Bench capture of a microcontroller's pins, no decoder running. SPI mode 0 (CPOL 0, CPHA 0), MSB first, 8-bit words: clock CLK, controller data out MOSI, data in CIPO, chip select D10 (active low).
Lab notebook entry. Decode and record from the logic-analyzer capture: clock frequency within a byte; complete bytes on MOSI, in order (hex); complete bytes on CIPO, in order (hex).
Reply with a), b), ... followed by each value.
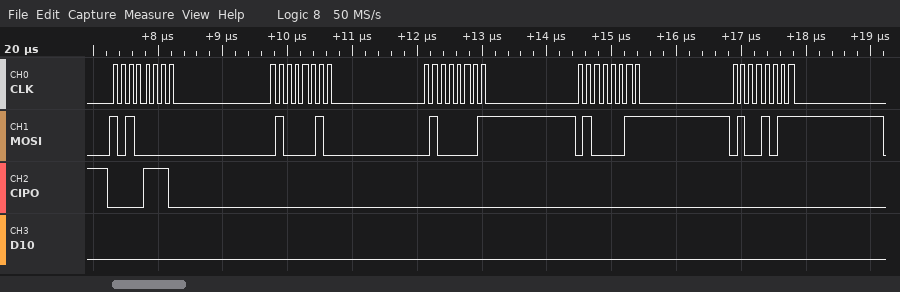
a) 8 MHz
b) A0 42 41 43 4B
c) 0E 00 00 00 00
